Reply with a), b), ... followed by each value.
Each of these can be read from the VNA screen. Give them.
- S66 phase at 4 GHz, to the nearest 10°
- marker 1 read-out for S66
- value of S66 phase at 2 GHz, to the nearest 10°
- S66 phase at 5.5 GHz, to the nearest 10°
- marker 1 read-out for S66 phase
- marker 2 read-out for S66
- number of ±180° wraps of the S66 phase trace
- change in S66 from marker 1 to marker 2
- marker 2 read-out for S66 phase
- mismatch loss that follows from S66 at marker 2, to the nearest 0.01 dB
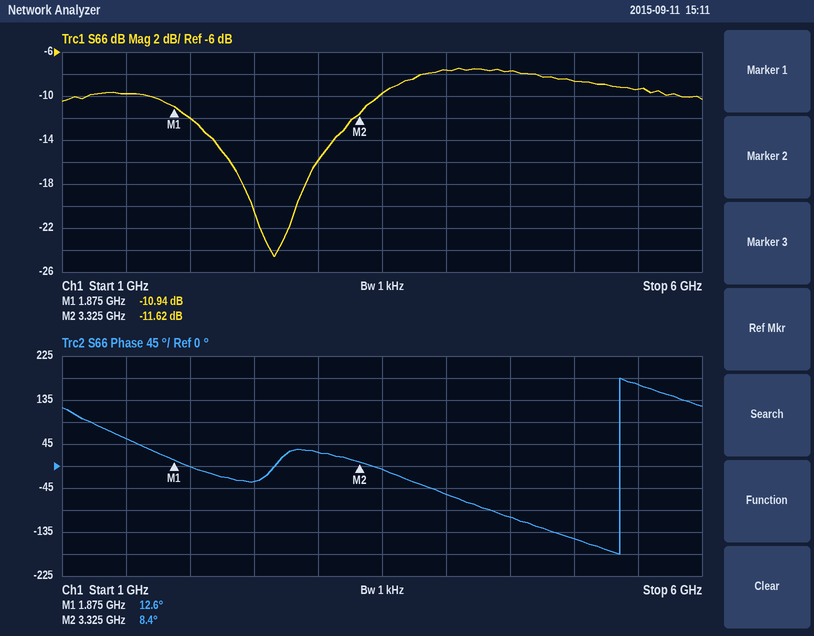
a) -60°
b) -10.94 dB
c) 0°
d) 170°
e) 12.6°
f) -11.62 dB
g) 1
h) -0.68 dB
i) 8.4°
j) 0.31 dB
